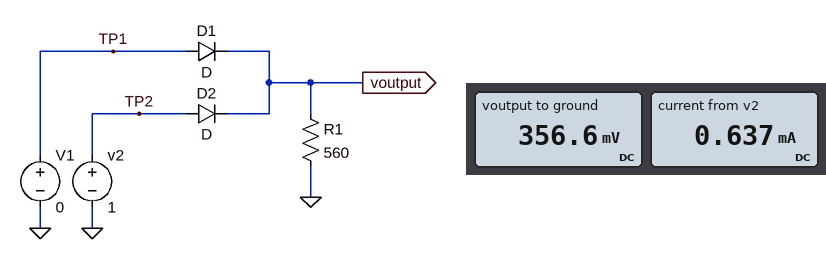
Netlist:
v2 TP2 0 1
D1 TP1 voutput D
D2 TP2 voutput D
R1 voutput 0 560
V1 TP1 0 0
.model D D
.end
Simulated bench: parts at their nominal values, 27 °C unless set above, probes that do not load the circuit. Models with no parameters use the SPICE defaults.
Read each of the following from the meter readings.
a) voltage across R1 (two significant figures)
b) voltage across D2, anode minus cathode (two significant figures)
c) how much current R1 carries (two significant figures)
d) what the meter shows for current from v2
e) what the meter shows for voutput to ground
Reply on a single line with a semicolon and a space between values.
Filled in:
360 mV; 640 mV; 640 µA; 0.637 mA; 356.6 mV
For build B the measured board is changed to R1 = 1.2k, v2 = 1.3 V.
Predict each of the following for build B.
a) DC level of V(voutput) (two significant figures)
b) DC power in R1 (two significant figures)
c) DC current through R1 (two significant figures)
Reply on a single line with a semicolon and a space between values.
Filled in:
660 mV; 360 µW; 550 µA
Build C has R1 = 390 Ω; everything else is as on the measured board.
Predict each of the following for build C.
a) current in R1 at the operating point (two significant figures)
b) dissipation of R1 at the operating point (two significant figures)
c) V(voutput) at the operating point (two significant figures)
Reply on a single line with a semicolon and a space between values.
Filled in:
890 µA; 310 µW; 350 mV
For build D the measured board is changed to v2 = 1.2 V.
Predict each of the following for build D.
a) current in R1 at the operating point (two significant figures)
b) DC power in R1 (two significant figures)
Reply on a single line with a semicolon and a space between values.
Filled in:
970 µA; 530 µW
